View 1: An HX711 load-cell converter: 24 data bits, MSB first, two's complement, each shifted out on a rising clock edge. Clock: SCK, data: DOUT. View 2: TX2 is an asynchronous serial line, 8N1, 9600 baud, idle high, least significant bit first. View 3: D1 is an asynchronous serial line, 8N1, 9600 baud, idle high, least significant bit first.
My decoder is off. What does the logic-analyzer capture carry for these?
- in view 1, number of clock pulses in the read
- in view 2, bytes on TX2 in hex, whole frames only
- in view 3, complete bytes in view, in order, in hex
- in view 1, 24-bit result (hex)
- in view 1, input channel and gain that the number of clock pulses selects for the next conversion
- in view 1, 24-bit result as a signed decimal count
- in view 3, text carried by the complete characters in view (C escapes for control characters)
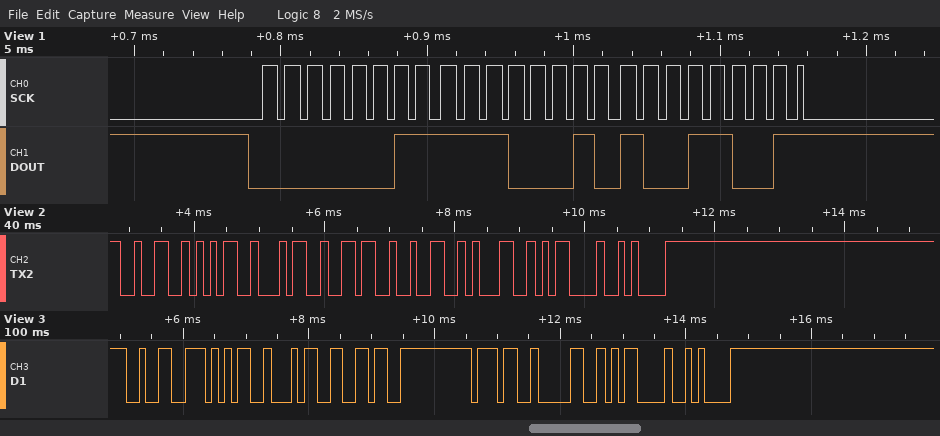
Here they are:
25
32 35 34 36 32 31 0D 0A
32 35 34 36 37 30 0D 0A
0x03E299
channel A, gain 128
254617
"254670\r\n"
